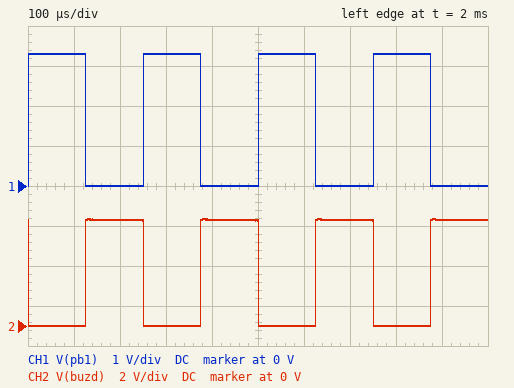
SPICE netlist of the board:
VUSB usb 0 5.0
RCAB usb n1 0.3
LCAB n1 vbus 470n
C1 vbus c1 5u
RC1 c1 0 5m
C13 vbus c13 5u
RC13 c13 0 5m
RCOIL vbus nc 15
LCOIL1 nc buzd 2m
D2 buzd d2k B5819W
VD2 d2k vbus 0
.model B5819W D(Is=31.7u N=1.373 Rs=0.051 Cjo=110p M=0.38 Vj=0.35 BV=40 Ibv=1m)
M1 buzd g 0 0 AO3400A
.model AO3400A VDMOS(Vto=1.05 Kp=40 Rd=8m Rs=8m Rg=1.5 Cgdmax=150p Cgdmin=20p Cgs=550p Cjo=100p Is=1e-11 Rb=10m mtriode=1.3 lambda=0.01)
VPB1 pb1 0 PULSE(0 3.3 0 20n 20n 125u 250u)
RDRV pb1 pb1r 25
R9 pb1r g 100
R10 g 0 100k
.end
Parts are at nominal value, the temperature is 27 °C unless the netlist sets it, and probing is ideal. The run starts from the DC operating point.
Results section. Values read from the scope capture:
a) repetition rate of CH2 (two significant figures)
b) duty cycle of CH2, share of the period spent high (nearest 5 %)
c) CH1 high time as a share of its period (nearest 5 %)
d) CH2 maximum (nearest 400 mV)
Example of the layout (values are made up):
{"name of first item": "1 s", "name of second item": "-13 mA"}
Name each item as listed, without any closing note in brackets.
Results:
{"repetition rate of CH2": "4.0 kHz", "duty cycle of CH2, share of the period spent high": "50 %", "CH1 high time as a share of its period": "50 %", "CH2 maximum": "5.2 V"}
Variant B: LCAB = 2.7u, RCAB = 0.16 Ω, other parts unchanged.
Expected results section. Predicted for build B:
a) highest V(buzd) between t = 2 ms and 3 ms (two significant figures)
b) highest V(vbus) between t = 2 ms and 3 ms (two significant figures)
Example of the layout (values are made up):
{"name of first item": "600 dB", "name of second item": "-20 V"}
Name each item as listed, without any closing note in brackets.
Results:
{"highest V(buzd) between t = 2 ms and 3 ms": "5.4 V", "highest V(vbus) between t = 2 ms and 3 ms": "5.1 V"}
